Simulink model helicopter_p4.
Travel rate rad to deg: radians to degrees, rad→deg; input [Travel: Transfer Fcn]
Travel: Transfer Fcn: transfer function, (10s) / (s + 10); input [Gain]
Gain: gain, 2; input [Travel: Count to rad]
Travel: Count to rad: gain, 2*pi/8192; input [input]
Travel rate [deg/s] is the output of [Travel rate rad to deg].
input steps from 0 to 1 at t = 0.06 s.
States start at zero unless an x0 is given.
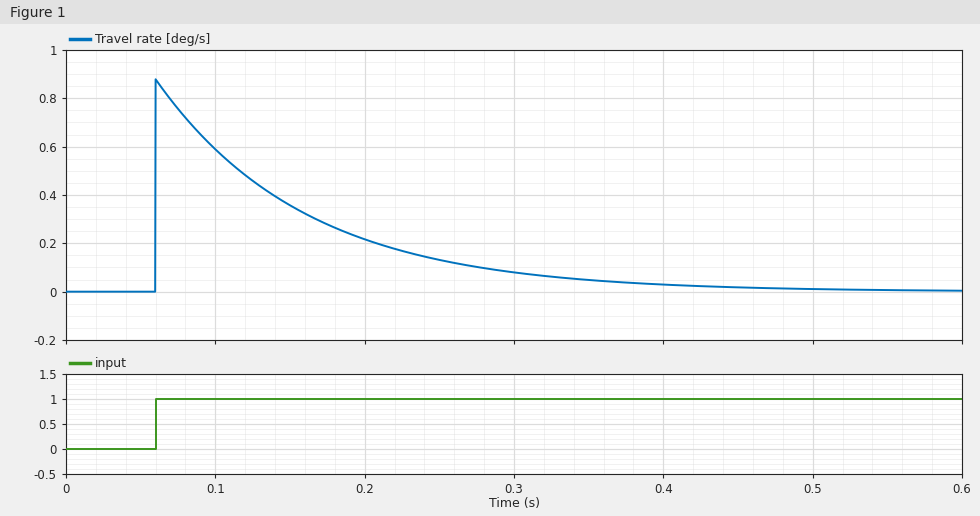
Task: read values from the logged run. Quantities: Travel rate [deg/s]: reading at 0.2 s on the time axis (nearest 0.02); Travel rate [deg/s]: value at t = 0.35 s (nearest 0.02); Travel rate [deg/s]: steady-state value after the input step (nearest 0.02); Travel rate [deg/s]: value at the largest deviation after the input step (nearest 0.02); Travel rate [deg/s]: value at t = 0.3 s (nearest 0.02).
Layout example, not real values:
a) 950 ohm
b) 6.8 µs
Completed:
a) 0.22
b) 0.04
c) 0.00
d) 0.88
e) 0.08
